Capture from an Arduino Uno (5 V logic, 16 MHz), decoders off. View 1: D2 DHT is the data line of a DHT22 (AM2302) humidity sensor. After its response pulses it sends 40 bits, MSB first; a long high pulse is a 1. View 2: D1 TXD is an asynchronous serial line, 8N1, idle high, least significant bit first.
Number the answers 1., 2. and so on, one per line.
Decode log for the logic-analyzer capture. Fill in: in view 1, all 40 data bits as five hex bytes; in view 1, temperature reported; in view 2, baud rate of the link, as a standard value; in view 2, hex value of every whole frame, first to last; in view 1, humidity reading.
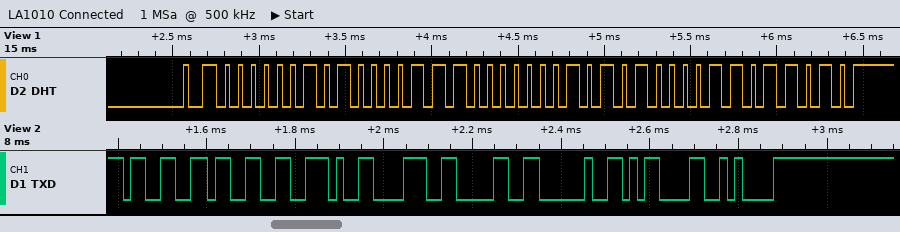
1. 02 87 01 50 DA
2. 33.6 °C
3. 57600 baud
4. 0x33 0x33 0x2E 0x38 0x30 0x20 0x0D 0x0A
5. 64.7 %
